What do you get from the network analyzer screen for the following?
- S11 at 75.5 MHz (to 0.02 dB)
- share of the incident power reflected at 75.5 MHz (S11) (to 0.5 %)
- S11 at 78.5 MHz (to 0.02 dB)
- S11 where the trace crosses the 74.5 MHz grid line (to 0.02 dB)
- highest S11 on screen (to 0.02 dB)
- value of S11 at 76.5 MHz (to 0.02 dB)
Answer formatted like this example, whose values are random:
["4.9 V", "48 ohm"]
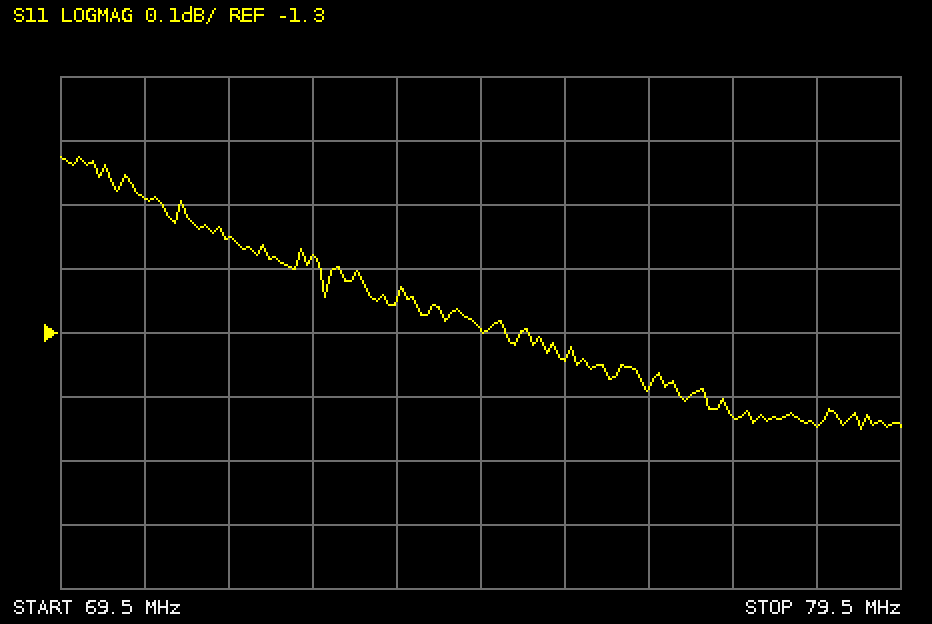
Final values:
["-1.34 dB", "73.5 %", "-1.44 dB", "-1.30 dB", "-1.02 dB", "-1.38 dB"]
